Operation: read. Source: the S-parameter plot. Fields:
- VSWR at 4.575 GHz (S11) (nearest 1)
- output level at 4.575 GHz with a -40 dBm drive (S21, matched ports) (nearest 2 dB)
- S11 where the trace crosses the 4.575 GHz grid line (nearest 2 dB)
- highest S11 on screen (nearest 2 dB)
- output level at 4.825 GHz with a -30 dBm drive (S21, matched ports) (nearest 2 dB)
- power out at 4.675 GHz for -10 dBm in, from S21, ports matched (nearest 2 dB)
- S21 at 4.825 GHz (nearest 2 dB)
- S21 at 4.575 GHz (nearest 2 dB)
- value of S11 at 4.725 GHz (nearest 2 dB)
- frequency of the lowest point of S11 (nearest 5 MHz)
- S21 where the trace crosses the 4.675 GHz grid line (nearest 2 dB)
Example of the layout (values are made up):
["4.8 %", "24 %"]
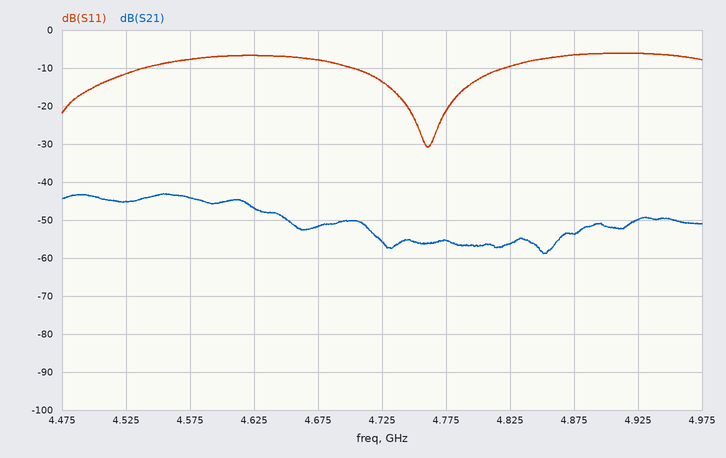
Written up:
["2", "-84 dBm", "-8 dB", "-6 dB", "-86 dBm", "-62 dBm", "-56 dB", "-44 dB", "-14 dB", "4.760 GHz", "-52 dB"]
